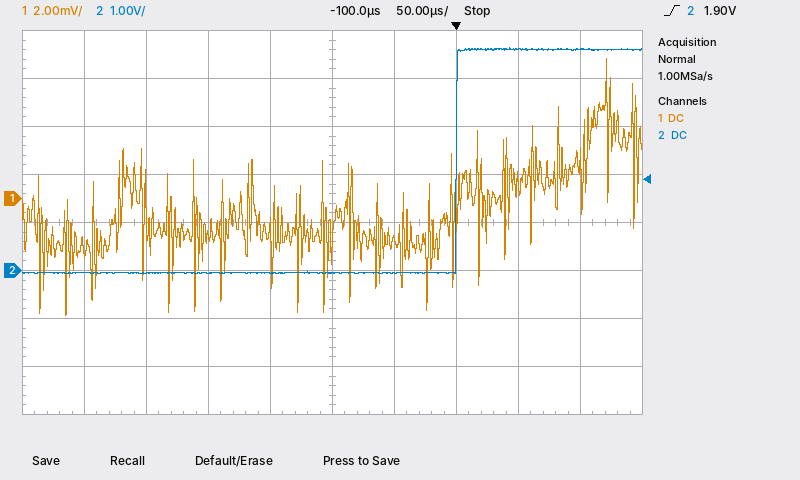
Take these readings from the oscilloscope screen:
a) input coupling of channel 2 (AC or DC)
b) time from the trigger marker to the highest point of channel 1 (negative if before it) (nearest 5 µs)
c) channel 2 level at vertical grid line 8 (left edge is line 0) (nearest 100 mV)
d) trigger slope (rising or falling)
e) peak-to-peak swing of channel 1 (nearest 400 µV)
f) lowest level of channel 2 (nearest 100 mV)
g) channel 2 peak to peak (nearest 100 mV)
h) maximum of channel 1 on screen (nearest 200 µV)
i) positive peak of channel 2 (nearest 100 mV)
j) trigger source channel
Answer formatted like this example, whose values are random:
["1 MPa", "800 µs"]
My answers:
["DC", "+120 µs", "4.6 V", "rising", "10.8 mV", "-100 mV", "4.7 V", "5.8 mV", "4.6 V", "channel 2"]
